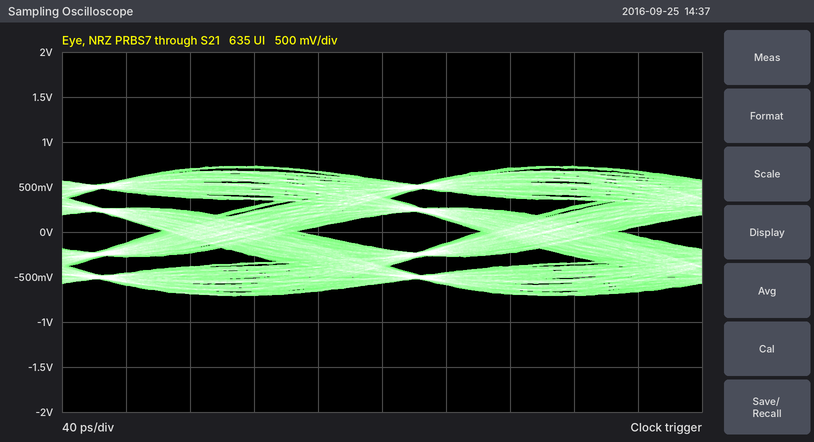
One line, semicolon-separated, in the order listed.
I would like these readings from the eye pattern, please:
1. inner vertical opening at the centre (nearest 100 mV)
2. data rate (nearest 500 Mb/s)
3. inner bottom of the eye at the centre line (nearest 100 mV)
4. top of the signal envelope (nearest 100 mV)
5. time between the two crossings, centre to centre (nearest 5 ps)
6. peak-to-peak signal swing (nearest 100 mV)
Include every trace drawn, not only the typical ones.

400 mV; 5.0 Gb/s; -200 mV; 700 mV; 200 ps; 1.4 V
